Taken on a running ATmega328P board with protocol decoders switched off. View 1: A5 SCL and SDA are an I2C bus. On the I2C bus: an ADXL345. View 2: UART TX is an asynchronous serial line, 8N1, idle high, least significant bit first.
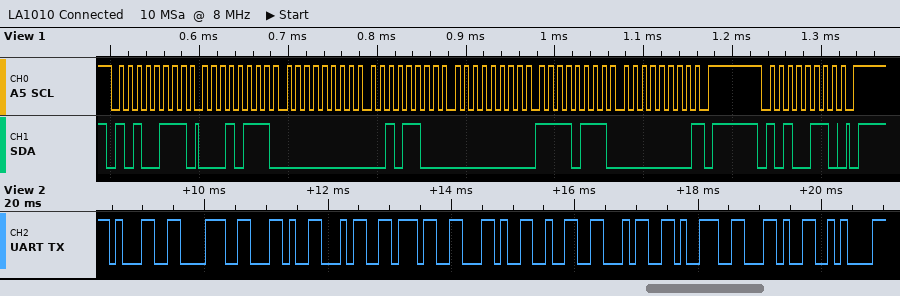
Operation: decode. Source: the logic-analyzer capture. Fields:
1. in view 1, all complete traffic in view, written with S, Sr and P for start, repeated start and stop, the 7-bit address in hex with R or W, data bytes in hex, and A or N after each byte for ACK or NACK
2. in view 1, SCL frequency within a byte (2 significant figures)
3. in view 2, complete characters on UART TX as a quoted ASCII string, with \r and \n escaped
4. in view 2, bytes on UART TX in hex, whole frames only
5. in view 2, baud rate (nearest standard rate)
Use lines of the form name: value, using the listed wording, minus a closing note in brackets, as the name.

in view 1, all complete traffic in view, written with S, Sr and P for start, repeated start and stop, the 7-bit address in hex with R or W, data bytes in hex, and A or N after each byte for ACK or NACK: S 53R A 17 A 00 A 2C A 00 A F7 A 00 N P S 53W A P
in view 1, SCL frequency within a byte: 100 kHz
in view 2, complete characters on UART TX as a quoted ASCII string, with \r and \n escaped: "18,47,249,\n"
in view 2, bytes on UART TX in hex, whole frames only: 0x31 0x38 0x2C 0x34 0x37 0x2C 0x32 0x34 0x39 0x2C 0x0A
in view 2, baud rate: 9600 baud
